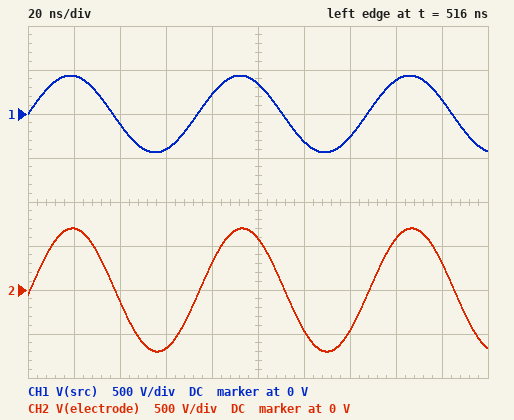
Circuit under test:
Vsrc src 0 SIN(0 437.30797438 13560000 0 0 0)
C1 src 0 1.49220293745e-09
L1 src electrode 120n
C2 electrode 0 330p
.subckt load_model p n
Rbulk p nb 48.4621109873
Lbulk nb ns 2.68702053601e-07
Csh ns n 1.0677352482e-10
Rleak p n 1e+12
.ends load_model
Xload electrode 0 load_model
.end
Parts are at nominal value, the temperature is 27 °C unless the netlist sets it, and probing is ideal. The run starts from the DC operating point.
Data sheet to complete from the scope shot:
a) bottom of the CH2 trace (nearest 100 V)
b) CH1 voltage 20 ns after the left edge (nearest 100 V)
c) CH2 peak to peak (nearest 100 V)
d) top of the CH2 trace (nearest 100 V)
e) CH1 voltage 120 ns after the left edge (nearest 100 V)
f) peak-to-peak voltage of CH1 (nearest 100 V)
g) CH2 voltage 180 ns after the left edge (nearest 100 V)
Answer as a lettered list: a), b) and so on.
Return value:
a) -700 V
b) 400 V
c) 1.4 kV
d) 700 V
e) -300 V
f) 900 V
g) 300 V
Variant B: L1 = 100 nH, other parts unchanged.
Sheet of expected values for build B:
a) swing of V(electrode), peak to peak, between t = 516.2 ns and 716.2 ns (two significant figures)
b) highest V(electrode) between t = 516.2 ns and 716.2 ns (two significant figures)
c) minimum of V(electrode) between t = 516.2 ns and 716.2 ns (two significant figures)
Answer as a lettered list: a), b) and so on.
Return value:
a) 1.3 kV
b) 640 V
c) -640 V
